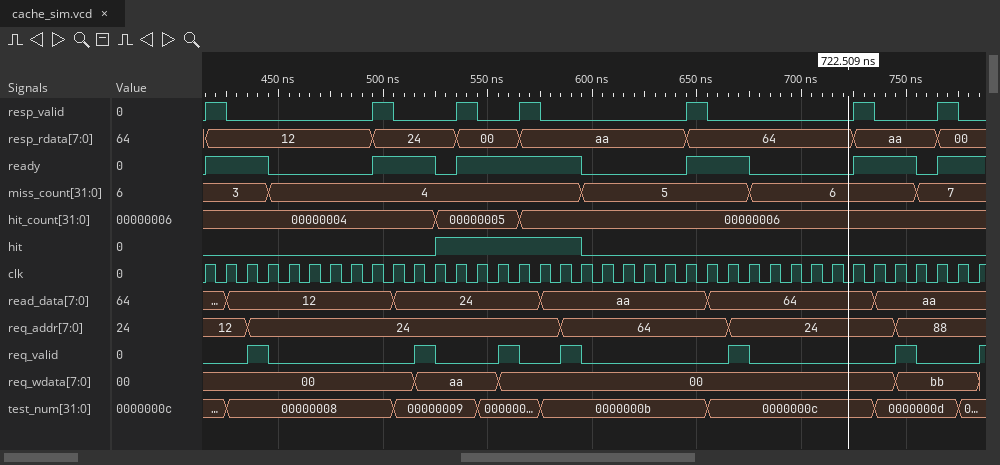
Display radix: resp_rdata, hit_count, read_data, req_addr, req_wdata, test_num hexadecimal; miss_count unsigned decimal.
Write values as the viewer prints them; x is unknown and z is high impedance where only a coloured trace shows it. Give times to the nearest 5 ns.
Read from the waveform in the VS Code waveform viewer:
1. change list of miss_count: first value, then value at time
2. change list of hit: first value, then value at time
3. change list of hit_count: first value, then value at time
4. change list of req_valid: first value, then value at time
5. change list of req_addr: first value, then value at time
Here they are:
3, 4 at 445 ns, 5 at 595 ns, 6 at 675 ns, 7 at 755 ns
0, 1 at 525 ns, 0 at 595 ns
00000004, 00000005 at 525 ns, 00000006 at 565 ns
0, 1 at 435 ns, 0 at 445 ns, 1 at 515 ns, 0 at 525 ns, 1 at 555 ns, 0 at 565 ns, 1 at 585 ns, 0 at 595 ns, 1 at 665 ns, 0 at 675 ns, 1 at 745 ns, 0 at 755 ns, 1 at 785 ns
12, 24 at 435 ns, 64 at 585 ns, 24 at 665 ns, 88 at 745 ns
